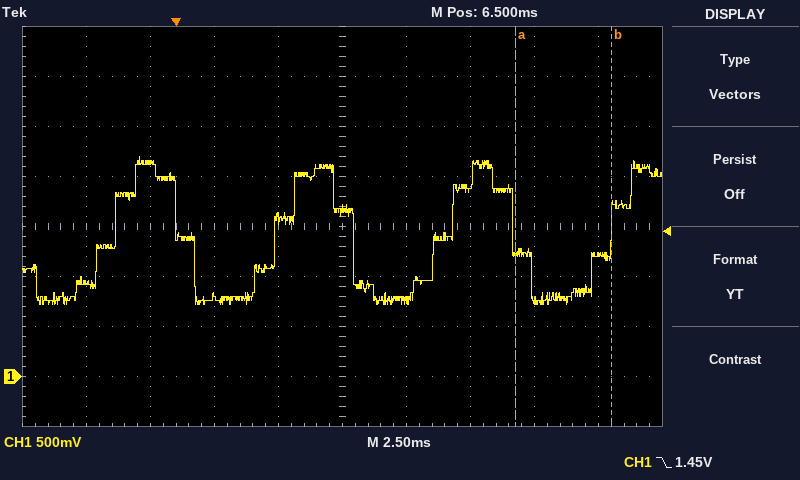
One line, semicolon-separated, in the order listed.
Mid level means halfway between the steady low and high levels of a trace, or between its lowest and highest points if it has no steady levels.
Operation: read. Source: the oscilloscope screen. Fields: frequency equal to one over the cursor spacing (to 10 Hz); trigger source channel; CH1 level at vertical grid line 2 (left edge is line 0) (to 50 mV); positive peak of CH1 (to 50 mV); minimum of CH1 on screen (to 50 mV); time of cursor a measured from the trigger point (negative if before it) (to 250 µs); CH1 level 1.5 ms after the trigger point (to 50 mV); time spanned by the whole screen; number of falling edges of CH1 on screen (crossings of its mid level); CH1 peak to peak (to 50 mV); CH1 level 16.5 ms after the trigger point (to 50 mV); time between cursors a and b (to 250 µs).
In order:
270 Hz; CH1; 2.15 V; 2.20 V; 700 mV; +13.25 ms; 800 mV; 25 ms; 3; 1.50 V; 1.20 V; 3.75 ms
